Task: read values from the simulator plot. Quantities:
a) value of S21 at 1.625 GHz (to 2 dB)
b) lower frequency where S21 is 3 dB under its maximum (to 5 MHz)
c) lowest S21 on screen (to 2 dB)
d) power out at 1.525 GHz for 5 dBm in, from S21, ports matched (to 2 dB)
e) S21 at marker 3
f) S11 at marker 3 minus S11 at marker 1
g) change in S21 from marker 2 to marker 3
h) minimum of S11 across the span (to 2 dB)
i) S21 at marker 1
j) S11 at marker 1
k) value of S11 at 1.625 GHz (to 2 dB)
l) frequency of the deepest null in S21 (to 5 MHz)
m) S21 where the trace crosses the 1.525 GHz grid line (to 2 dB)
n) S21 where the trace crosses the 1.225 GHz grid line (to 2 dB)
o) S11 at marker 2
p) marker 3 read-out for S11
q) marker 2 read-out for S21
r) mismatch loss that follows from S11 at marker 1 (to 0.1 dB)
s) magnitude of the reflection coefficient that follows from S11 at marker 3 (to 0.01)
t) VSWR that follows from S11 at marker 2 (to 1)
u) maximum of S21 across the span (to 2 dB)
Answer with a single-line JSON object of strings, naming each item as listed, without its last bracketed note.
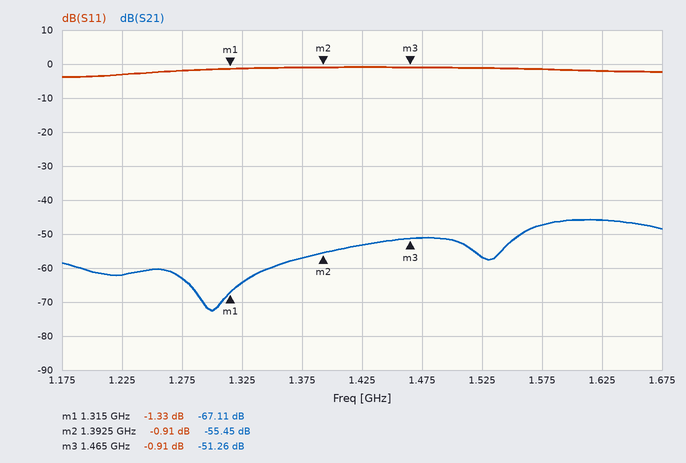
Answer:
{"value of S21 at 1.625 GHz": "-46 dB", "lower frequency where S21 is 3 dB under its maximum": "1.565 GHz", "lowest S21 on screen": "-72 dB", "power out at 1.525 GHz for 5 dBm in, from S21, ports matched": "-52 dBm", "S21 at marker 3": "-51.26 dB", "S11 at marker 3 minus S11 at marker 1": "0.42 dB", "change in S21 from marker 2 to marker 3": "4.19 dB", "minimum of S11 across the span": "-4 dB", "S21 at marker 1": "-67.11 dB", "S11 at marker 1": "-1.33 dB", "value of S11 at 1.625 GHz": "-2 dB", "frequency of the deepest null in S21": "1.300 GHz", "S21 where the trace crosses the 1.525 GHz grid line": "-56 dB", "S21 where the trace crosses the 1.225 GHz grid line": "-62 dB", "S11 at marker 2": "-0.91 dB", "marker 3 read-out for S11": "-0.91 dB", "marker 2 read-out for S21": "-55.45 dB", "mismatch loss that follows from S11 at marker 1": "5.8 dB", "magnitude of the reflection coefficient that follows from S11 at marker 3": "0.90", "VSWR that follows from S11 at marker 2": "19", "maximum of S21 across the span": "-46 dB"}
